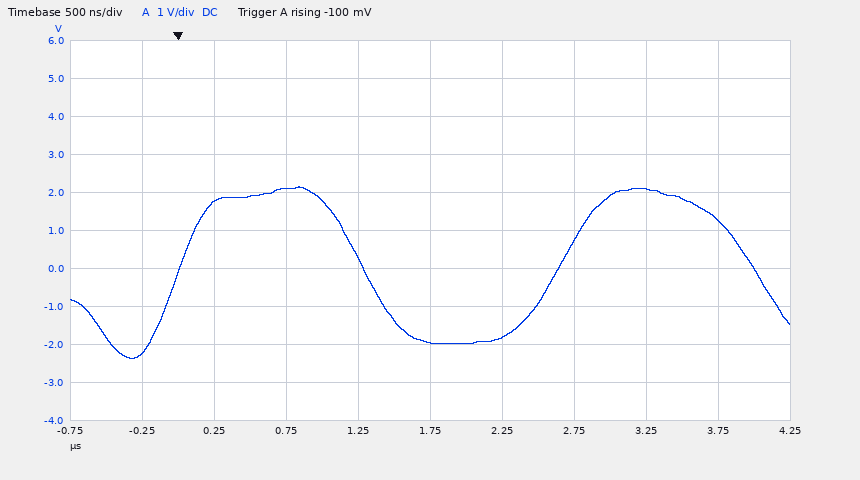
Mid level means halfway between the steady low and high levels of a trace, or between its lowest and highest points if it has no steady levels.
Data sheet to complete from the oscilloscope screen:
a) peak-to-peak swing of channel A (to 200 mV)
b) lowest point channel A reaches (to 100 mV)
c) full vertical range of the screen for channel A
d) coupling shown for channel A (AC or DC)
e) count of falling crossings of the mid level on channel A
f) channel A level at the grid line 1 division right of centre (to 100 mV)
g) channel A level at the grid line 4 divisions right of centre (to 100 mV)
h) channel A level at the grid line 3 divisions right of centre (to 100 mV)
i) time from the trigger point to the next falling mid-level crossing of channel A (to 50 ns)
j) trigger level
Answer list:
4.6 V
-2.4 V
10 V
DC
2
-1.8 V
1.3 V
2.1 V
1.30 µs
-100 mV
